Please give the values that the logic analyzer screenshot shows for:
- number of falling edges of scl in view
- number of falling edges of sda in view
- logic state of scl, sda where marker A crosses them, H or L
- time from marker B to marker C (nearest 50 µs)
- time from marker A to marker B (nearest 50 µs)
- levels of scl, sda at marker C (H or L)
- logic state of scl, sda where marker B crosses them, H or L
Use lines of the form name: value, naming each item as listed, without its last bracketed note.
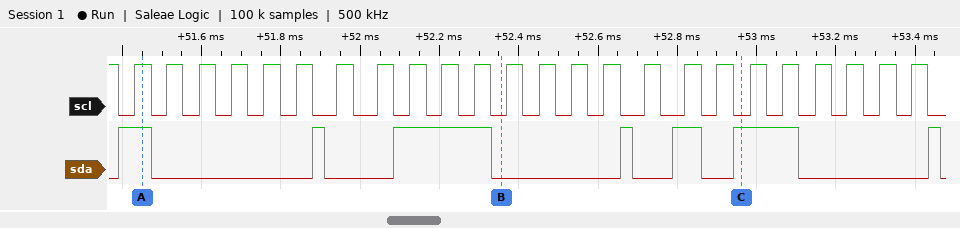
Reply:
number of falling edges of scl in view: 25
number of falling edges of sda in view: 7
logic state of scl, sda where marker A crosses them, H or L: scl=H, sda=H
time from marker B to marker C: 600 µs
time from marker A to marker B: 900 µs
levels of scl, sda at marker C: scl=L, sda=H
logic state of scl, sda where marker B crosses them, H or L: scl=L, sda=L
